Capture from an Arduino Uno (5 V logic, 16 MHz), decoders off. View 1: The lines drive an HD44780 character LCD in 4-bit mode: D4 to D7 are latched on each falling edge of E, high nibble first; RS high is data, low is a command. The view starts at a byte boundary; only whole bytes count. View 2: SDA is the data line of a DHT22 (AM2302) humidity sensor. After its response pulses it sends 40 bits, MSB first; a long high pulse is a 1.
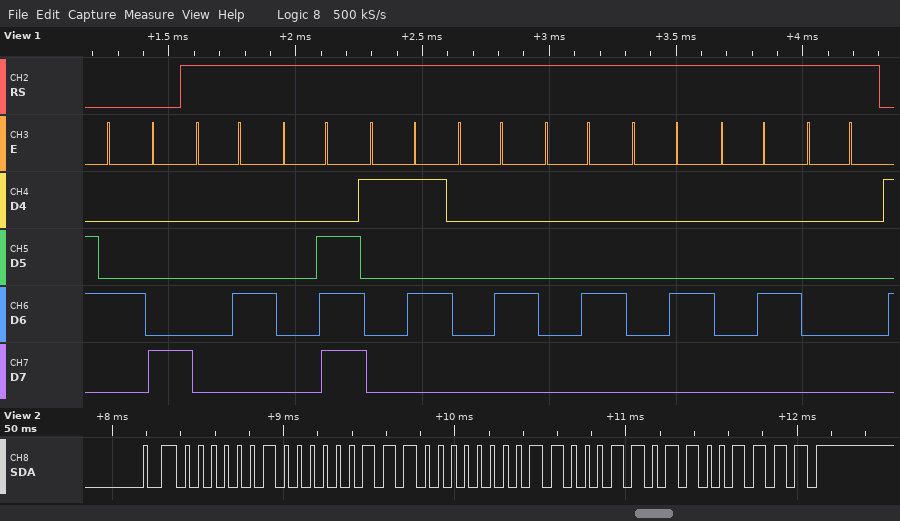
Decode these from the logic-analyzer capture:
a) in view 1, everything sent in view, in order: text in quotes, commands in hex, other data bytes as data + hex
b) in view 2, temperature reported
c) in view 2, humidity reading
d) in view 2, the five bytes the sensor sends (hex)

0x48 data 04 0E 15 04 04 04 04 00
19.8 °C
51.9 %
02 07 00 C6 CF
